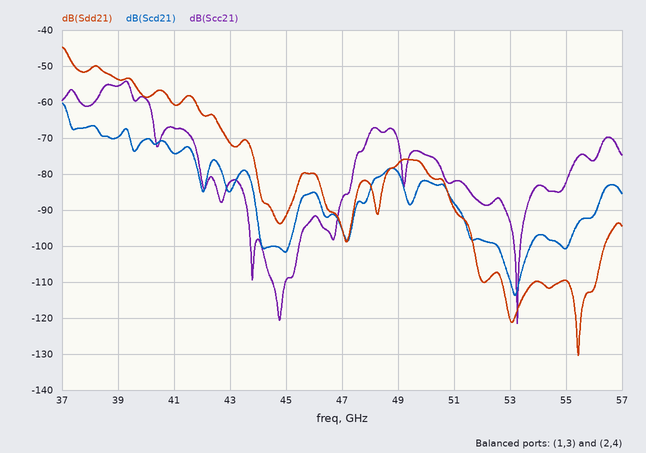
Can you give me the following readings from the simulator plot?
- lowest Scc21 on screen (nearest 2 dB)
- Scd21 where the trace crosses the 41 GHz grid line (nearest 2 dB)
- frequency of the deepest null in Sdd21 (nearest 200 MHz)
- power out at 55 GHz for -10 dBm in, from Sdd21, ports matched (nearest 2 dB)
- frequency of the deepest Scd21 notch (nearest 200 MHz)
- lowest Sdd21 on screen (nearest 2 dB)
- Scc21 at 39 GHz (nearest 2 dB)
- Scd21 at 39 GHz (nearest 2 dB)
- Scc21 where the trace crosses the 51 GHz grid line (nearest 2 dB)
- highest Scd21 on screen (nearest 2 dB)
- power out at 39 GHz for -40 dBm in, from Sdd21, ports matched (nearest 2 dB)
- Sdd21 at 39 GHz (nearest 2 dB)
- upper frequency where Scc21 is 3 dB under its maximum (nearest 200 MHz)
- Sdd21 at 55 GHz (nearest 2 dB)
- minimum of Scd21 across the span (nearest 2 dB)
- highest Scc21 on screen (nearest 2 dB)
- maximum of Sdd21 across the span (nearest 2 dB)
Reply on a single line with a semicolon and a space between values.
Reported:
-122 dB; -74 dB; 55.4 GHz; -120 dBm; 53.2 GHz; -130 dB; -56 dB; -70 dB; -82 dB; -60 dB; -94 dBm; -54 dB; 39.4 GHz; -110 dB; -114 dB; -54 dB; -44 dB
